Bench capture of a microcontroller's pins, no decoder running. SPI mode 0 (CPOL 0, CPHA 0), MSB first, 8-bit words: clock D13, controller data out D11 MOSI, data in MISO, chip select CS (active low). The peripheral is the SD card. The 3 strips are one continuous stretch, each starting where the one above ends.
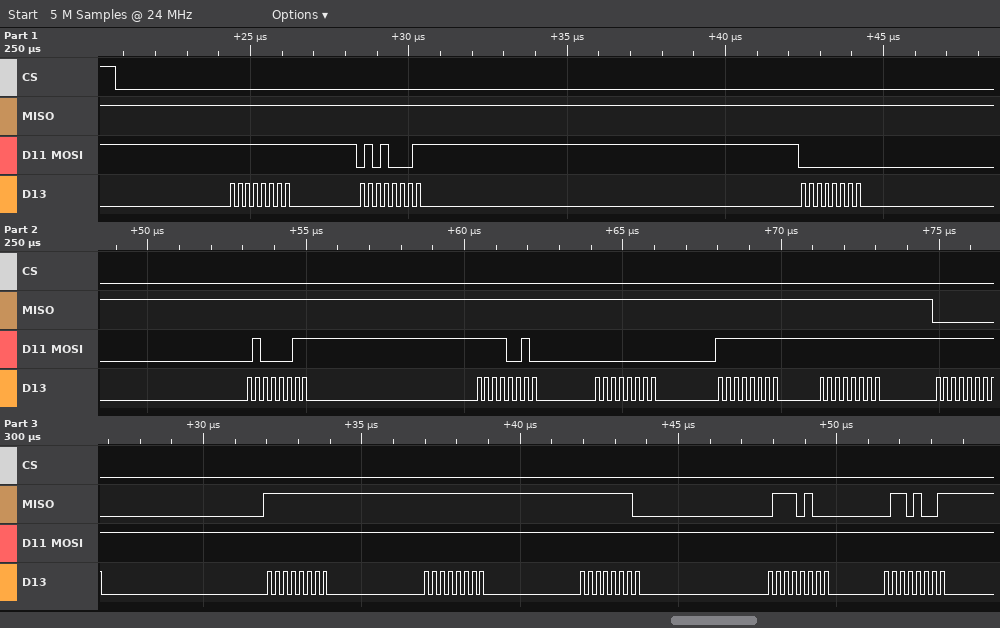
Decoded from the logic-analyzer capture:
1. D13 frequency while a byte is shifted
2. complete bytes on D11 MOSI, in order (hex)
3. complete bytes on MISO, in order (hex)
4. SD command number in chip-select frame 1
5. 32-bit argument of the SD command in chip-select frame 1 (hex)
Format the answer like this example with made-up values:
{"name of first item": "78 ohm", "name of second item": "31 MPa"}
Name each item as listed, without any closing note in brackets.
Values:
{"D13 frequency while a byte is shifted": "4 MHz", "complete bytes on D11 MOSI, in order": "FF 51 00 43 F2 00 FF FF FF FF FF FF FF FF", "complete bytes on MISO, in order": "FF FF FF FF FF FF FF FF 00 FF FF FE 74 69", "SD command number in chip-select frame 1": "CMD17", "32-bit argument of the SD command in chip-select frame 1": "0x0043F200"}
